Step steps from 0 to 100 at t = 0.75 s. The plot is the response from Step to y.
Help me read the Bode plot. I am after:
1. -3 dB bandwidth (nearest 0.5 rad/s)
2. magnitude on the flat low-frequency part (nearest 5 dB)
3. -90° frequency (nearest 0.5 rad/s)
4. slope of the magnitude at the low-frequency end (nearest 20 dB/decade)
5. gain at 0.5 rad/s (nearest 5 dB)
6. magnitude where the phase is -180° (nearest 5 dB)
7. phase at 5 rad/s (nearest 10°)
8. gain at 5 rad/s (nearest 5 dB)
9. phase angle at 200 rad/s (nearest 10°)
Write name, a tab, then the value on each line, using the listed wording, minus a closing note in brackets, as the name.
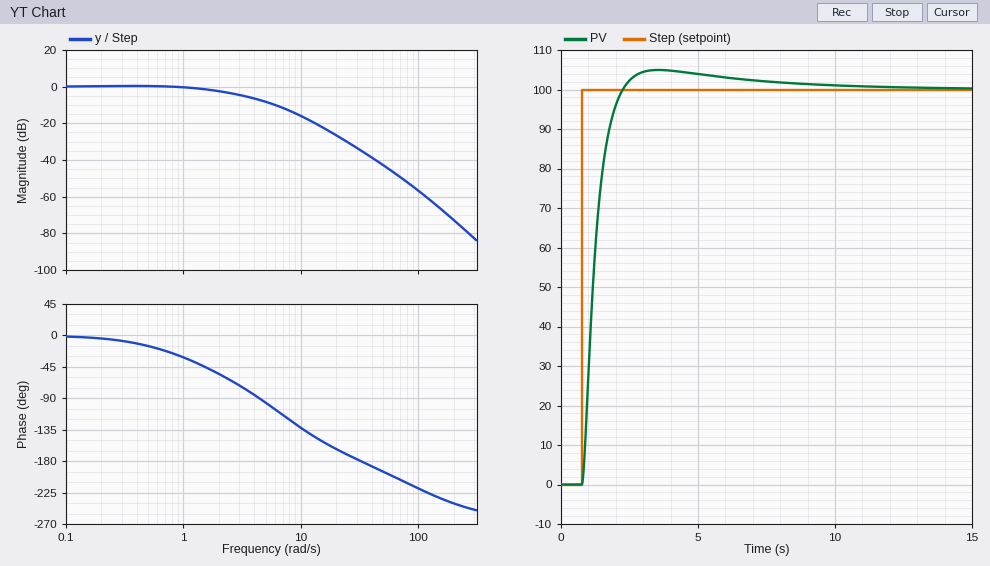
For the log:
-3 dB bandwidth	2.0 rad/s
magnitude on the flat low-frequency part	0 dB
-90° frequency	4.5 rad/s
slope of the magnitude at the low-frequency end	0 dB/decade
gain at 0.5 rad/s	0 dB
magnitude where the phase is -180°	-35 dB
phase at 5 rad/s	-100°
gain at 5 rad/s	-10 dB
phase angle at 200 rad/s	-240°
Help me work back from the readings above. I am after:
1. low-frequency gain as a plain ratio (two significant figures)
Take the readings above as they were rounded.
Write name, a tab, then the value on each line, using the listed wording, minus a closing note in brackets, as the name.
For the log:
low-frequency gain as a plain ratio	1.0
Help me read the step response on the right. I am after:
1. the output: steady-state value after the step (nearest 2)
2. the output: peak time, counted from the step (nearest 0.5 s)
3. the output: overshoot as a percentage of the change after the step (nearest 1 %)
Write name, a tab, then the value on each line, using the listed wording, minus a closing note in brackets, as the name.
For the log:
the output: steady-state value after the step	100
the output: peak time, counted from the step	3.0 s
the output: overshoot as a percentage of the change after the step	5 %
